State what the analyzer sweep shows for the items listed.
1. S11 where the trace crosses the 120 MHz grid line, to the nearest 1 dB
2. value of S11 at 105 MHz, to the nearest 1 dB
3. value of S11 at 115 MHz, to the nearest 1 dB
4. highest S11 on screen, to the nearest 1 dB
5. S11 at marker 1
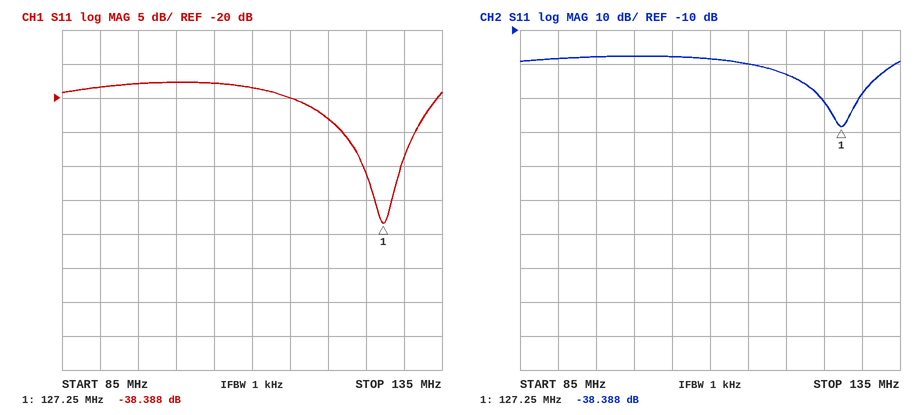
-23 dB
-18 dB
-20 dB
-18 dB
-38.388 dB
